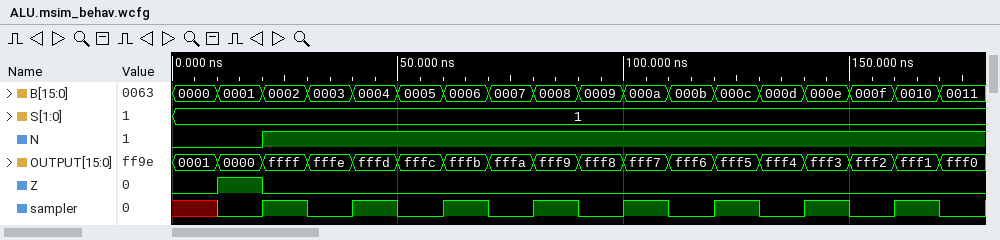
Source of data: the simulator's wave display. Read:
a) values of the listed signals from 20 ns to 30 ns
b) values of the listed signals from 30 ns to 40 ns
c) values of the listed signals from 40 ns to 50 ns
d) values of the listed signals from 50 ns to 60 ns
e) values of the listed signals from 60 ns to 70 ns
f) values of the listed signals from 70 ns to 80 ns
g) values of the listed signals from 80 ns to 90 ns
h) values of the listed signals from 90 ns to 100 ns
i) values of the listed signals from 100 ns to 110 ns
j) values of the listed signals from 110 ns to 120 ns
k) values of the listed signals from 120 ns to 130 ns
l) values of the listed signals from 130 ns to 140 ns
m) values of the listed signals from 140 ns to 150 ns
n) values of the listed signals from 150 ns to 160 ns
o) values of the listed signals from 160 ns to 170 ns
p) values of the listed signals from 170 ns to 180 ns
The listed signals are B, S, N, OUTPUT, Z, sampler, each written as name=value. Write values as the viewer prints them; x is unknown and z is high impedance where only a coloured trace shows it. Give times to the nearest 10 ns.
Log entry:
B=0002, S=1, N=1, OUTPUT=ffff, Z=0, sampler=1
B=0003, S=1, N=1, OUTPUT=fffe, Z=0, sampler=0
B=0004, S=1, N=1, OUTPUT=fffd, Z=0, sampler=1
B=0005, S=1, N=1, OUTPUT=fffc, Z=0, sampler=0
B=0006, S=1, N=1, OUTPUT=fffb, Z=0, sampler=1
B=0007, S=1, N=1, OUTPUT=fffa, Z=0, sampler=0
B=0008, S=1, N=1, OUTPUT=fff9, Z=0, sampler=1
B=0009, S=1, N=1, OUTPUT=fff8, Z=0, sampler=0
B=000a, S=1, N=1, OUTPUT=fff7, Z=0, sampler=1
B=000b, S=1, N=1, OUTPUT=fff6, Z=0, sampler=0
B=000c, S=1, N=1, OUTPUT=fff5, Z=0, sampler=1
B=000d, S=1, N=1, OUTPUT=fff4, Z=0, sampler=0
B=000e, S=1, N=1, OUTPUT=fff3, Z=0, sampler=1
B=000f, S=1, N=1, OUTPUT=fff2, Z=0, sampler=0
B=0010, S=1, N=1, OUTPUT=fff1, Z=0, sampler=1
B=0011, S=1, N=1, OUTPUT=fff0, Z=0, sampler=0
